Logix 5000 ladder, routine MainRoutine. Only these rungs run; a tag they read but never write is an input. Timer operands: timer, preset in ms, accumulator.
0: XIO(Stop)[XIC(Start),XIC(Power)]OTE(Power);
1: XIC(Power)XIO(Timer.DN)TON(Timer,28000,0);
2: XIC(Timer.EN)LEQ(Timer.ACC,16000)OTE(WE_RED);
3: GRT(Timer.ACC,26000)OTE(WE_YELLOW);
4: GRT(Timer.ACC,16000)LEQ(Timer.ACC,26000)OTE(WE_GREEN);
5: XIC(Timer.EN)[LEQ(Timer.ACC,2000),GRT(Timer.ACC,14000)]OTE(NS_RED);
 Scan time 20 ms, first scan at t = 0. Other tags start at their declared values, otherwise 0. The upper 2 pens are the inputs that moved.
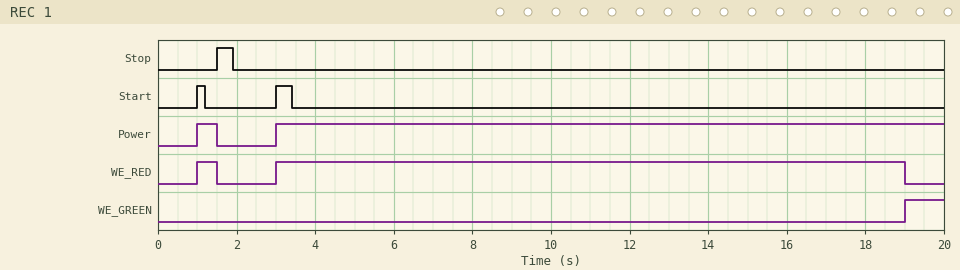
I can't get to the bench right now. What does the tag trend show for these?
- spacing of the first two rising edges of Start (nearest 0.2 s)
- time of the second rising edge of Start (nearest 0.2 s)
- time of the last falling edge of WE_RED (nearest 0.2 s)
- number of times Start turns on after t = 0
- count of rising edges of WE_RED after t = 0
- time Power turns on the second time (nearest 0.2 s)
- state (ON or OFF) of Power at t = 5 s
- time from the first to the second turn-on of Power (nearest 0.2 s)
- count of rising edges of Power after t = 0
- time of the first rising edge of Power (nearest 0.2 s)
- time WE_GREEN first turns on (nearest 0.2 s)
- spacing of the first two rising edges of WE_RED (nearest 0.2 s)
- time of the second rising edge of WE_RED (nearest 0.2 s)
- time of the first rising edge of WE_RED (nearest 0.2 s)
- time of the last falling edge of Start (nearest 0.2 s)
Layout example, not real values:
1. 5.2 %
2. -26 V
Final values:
1. 2.0 s
2. 3.0 s
3. 19.0 s
4. 2
5. 2
6. 3.0 s
7. ON
8. 2.0 s
9. 2
10. 1.0 s
11. 19.0 s
12. 2.0 s
13. 3.0 s
14. 1.0 s
15. 3.4 s
